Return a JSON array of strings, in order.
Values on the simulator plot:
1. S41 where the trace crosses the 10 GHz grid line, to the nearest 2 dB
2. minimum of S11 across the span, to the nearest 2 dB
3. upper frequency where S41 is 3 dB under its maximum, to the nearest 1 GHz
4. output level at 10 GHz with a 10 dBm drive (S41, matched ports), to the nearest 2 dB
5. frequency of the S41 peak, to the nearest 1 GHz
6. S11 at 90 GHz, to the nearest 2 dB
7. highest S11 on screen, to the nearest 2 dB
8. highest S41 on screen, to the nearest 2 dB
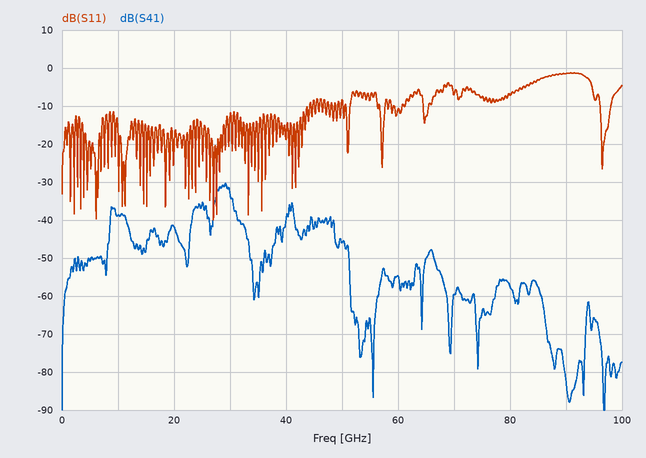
["-38 dB", "-40 dB", "30 GHz", "-28 dBm", "29 GHz", "-2 dB", "-2 dB", "-30 dB"]
